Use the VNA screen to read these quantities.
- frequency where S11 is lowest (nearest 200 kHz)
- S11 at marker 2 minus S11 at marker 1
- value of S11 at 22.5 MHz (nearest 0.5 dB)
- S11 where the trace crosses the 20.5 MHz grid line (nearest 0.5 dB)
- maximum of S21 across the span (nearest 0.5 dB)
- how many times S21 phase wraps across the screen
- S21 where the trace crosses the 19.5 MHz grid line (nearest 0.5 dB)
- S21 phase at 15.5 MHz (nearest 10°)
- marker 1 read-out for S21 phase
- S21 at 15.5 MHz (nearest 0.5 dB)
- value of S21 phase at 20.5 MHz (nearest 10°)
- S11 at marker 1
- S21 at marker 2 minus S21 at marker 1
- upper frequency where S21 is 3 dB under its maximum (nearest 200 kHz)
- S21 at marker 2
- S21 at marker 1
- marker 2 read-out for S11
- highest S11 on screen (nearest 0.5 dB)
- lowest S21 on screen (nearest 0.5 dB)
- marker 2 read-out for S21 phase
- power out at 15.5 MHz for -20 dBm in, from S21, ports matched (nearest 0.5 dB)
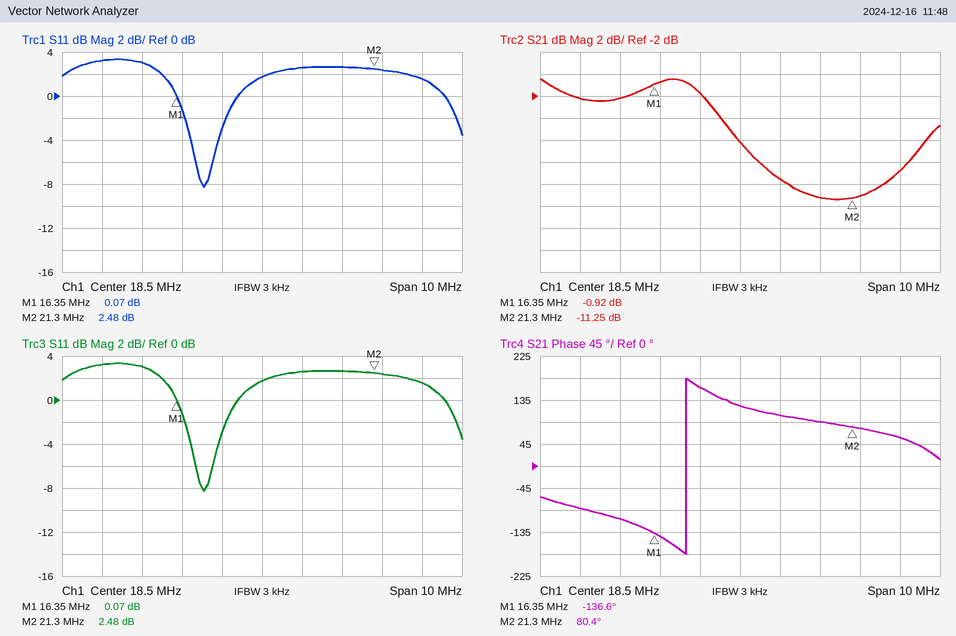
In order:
17.0 MHz
2.41 dB
1.5 dB
2.5 dB
-0.5 dB
1
-9.5 dB
-110°
-136.6°
-2.0 dB
90°
0.07 dB
-10.33 dB
17.8 MHz
-11.25 dB
-0.92 dB
2.48 dB
3.5 dB
-11.5 dB
80.4°
-22.0 dBm
